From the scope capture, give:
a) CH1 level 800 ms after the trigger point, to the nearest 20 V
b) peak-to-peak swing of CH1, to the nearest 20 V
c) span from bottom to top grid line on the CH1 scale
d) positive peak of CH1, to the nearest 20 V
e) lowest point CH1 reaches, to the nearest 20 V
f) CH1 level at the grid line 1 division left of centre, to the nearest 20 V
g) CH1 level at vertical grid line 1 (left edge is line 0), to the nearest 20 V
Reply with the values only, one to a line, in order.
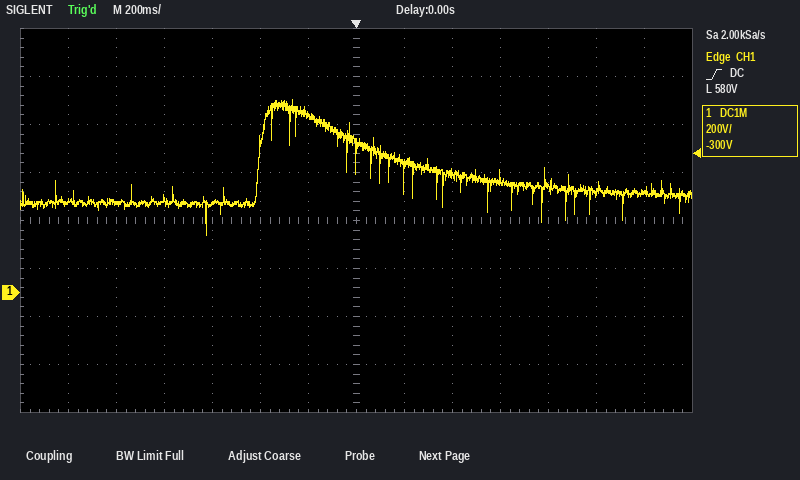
440 V
560 V
1.6 kV
800 V
240 V
740 V
380 V
